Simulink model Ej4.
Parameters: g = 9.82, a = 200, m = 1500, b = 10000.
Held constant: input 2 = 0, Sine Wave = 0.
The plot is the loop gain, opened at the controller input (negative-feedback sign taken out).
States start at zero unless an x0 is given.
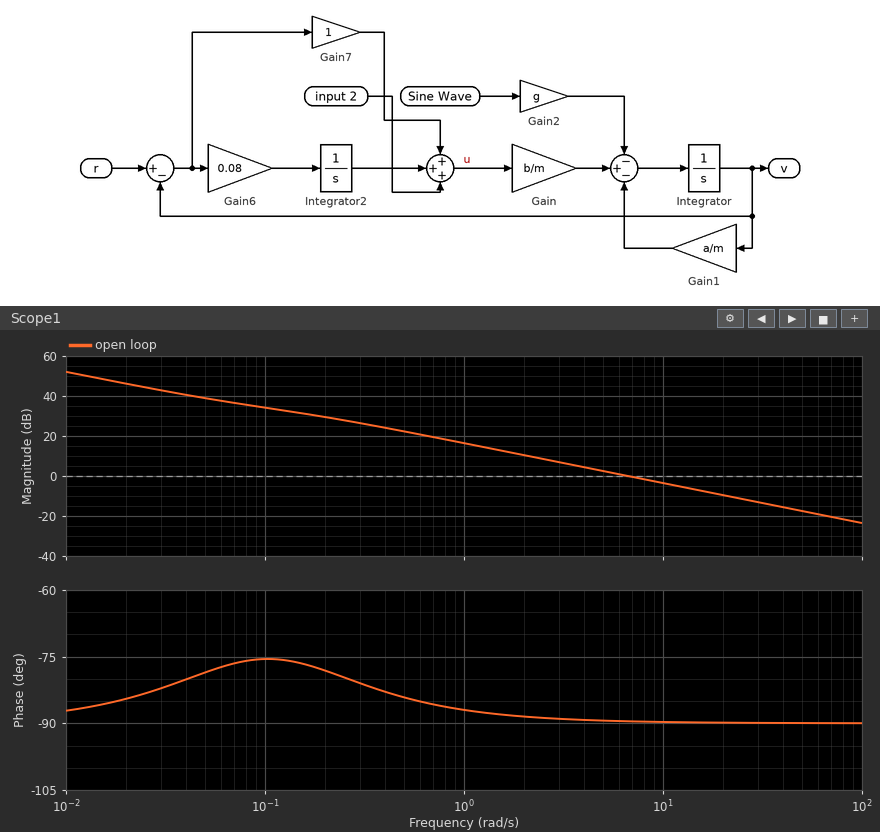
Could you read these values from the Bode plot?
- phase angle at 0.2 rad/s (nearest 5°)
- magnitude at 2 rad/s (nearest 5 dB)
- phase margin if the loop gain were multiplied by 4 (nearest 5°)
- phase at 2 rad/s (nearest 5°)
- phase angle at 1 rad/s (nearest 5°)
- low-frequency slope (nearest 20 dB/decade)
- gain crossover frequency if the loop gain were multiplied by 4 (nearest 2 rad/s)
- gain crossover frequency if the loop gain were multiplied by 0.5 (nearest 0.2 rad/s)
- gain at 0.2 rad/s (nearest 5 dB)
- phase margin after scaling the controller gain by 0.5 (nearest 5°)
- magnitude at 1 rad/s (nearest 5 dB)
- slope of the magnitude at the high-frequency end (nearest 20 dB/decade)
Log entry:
-80°
10 dB
90°
-90°
-85°
-20 dB/decade
26 rad/s
3.4 rad/s
30 dB
90°
15 dB
-20 dB/decade
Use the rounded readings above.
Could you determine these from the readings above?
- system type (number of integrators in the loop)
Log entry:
1
